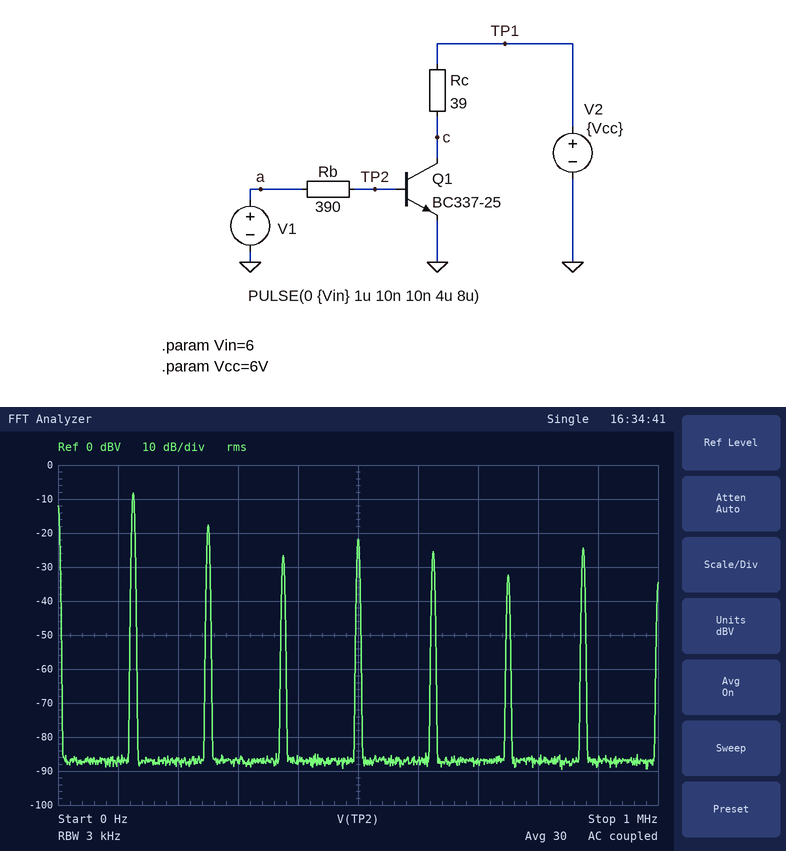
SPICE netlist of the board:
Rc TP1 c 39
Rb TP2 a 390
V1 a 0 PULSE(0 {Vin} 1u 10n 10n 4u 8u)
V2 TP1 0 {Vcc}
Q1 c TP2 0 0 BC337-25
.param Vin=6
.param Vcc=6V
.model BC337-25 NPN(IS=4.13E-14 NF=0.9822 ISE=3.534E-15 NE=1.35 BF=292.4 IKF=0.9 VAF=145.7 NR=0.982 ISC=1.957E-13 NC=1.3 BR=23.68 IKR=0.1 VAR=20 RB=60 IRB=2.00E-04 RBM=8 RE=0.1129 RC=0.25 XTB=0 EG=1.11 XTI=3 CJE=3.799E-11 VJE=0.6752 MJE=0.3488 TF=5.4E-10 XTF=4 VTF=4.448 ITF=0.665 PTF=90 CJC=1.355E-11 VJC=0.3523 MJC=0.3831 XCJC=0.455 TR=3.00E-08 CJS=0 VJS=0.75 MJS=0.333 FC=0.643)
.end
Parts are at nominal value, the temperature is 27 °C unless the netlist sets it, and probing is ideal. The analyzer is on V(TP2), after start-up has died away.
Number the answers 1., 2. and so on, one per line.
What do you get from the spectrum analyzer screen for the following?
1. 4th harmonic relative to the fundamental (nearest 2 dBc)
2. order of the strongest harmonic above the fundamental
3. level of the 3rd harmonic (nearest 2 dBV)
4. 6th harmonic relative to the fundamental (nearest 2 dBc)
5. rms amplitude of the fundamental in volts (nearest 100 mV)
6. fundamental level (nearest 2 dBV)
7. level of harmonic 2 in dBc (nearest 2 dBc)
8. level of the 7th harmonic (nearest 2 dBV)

1. -14 dBc
2. 2
3. -26 dBV
4. -24 dBc
5. 400 mV
6. -8 dBV
7. -10 dBc
8. -24 dBV
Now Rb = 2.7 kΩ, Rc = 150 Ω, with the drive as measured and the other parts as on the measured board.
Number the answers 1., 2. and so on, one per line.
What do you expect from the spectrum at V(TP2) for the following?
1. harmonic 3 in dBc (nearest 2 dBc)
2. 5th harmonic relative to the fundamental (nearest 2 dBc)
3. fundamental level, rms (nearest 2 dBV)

1. -28 dBc
2. -14 dBc
3. -10 dBV
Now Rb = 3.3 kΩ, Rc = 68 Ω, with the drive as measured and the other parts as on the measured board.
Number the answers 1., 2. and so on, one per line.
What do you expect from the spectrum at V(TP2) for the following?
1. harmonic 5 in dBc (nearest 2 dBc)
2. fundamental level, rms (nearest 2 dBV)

1. -20 dBc
2. -10 dBV
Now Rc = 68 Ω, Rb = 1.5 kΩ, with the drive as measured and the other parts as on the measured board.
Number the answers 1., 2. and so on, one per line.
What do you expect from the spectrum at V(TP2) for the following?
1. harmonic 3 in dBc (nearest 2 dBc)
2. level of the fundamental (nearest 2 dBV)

1. -20 dBc
2. -10 dBV
